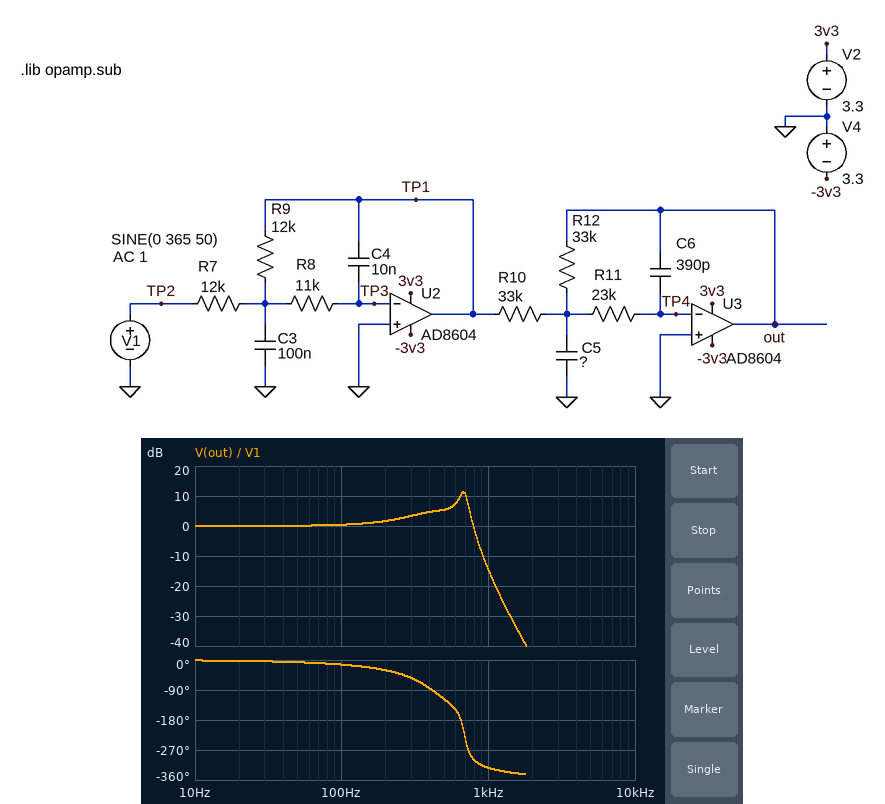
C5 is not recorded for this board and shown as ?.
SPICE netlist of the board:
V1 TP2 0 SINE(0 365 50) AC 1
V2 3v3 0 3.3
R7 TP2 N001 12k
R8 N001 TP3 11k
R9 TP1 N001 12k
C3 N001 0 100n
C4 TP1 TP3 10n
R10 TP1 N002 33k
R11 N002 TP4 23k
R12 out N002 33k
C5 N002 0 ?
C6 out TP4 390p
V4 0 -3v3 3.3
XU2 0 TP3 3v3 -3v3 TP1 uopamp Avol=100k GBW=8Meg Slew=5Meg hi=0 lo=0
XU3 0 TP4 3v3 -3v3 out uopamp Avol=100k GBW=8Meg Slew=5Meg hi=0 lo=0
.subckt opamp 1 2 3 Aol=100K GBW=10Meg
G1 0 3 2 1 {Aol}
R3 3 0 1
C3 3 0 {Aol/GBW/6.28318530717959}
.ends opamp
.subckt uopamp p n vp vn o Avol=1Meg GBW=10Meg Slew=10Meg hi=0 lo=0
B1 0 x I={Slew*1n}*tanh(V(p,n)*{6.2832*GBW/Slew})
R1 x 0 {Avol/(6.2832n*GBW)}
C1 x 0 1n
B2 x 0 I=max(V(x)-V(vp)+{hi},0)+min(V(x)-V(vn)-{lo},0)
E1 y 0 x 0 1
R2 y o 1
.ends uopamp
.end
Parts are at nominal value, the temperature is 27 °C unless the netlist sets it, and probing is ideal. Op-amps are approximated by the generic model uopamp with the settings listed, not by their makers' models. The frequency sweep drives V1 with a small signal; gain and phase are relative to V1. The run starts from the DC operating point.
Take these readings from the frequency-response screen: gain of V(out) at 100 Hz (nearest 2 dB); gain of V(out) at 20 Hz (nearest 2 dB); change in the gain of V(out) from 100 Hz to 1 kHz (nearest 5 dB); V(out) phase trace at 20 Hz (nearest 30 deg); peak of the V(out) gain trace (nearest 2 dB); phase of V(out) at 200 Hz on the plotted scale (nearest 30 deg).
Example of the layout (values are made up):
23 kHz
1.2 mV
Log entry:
0 dB
0 dB
-15 dB
0 deg
12 dB
-30 deg
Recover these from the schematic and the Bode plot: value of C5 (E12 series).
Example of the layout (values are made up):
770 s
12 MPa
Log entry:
180 nF
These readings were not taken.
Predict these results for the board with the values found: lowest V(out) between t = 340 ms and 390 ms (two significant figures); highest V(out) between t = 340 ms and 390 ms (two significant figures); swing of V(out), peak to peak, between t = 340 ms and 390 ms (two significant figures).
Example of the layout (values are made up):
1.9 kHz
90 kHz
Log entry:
-3.3 V
3.3 V
6.6 V
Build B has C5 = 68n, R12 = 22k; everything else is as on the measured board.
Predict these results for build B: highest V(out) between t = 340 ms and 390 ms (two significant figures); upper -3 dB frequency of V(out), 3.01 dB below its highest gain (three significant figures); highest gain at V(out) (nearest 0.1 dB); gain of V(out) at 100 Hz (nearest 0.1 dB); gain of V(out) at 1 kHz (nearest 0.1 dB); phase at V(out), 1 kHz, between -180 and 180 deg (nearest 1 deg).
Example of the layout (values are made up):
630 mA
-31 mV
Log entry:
3.3 V
549 Hz
-1.3 dB
-3.2 dB
-10.8 dB
-171 deg
